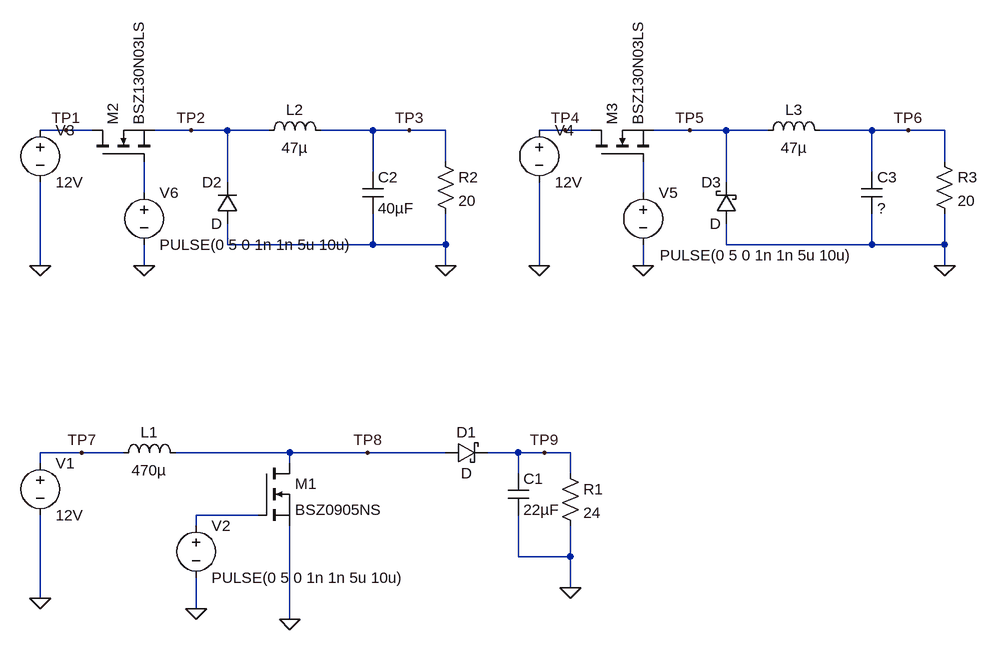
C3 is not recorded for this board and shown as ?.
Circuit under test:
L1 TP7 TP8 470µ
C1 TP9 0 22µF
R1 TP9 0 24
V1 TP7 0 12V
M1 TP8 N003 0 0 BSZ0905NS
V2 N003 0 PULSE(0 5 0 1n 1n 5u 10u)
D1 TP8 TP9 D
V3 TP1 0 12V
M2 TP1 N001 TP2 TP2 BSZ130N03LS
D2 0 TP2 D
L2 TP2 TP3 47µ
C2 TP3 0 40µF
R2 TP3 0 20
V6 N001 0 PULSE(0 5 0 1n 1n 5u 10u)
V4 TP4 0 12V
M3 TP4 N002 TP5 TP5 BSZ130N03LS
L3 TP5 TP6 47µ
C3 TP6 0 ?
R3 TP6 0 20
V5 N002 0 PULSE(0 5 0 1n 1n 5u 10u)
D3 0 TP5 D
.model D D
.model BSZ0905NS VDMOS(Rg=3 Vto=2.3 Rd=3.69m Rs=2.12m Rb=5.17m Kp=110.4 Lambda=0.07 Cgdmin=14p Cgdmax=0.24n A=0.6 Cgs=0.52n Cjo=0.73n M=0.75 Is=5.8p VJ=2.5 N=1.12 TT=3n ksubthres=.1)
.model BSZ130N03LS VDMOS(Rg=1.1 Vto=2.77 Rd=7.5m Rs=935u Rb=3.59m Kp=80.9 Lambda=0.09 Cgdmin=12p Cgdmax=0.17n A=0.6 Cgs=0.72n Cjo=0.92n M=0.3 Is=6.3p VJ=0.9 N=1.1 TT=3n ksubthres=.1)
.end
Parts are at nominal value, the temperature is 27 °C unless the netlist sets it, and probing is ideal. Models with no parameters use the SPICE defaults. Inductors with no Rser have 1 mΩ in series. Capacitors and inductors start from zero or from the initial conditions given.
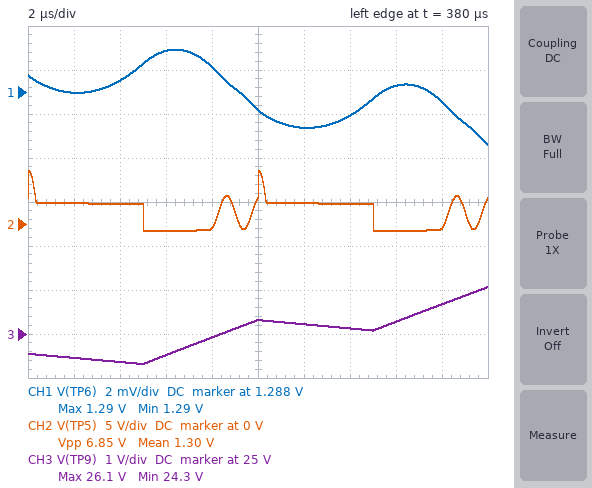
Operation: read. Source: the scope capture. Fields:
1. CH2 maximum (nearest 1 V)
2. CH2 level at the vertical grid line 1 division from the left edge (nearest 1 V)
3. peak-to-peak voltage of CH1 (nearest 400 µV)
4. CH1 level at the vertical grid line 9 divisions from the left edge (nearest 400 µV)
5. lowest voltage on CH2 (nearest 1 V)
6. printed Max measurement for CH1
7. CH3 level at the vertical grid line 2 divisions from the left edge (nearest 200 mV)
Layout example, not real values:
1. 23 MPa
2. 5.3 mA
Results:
1. 6 V
2. 2 V
3. 4.4 mV
4. 1.2876 V
5. -1 V
6. 1.29 V
7. 24.4 V
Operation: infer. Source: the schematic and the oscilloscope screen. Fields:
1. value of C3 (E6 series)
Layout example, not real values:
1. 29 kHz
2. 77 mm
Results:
1. 68 µF
